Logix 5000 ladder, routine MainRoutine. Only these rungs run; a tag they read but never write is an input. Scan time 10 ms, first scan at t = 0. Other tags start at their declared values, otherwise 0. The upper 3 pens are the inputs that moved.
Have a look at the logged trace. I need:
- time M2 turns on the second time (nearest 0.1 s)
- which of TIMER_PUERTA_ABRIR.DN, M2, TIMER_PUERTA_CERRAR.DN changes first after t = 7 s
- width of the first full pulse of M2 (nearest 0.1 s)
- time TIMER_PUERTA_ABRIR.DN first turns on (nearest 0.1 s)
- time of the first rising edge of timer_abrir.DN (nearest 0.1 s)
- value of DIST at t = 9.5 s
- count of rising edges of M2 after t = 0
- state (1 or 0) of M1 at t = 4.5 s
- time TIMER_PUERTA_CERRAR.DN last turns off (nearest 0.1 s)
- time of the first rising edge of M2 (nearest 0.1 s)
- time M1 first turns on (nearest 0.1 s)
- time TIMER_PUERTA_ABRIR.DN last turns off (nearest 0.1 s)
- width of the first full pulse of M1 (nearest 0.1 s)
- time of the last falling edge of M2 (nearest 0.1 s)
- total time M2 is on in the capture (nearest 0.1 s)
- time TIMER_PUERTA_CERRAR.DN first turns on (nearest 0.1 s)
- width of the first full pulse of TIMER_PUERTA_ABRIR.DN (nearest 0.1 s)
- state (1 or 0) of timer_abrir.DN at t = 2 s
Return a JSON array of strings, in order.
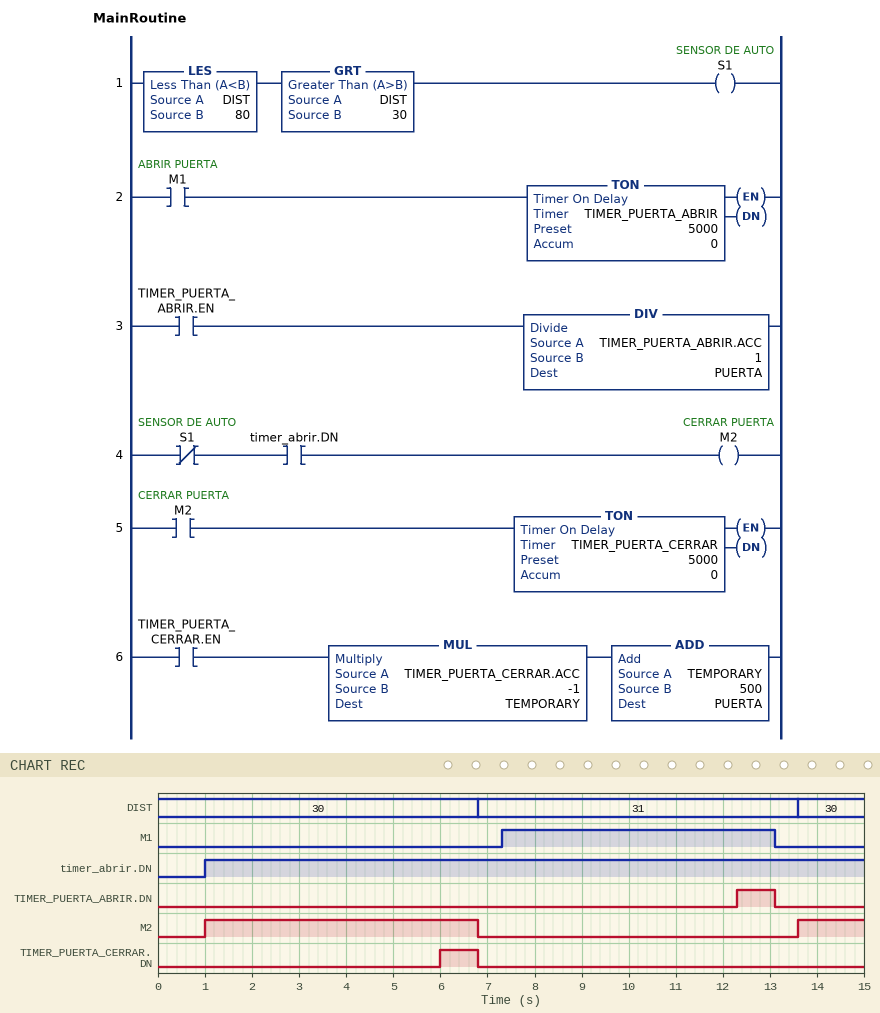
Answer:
["13.6 s", "TIMER_PUERTA_ABRIR.DN", "5.8 s", "12.3 s", "1.0 s", "31", "2", "0", "6.8 s", "1.0 s", "7.3 s", "13.1 s", "5.8 s", "6.8 s", "7.2 s", "6.0 s", "0.8 s", "1"]
